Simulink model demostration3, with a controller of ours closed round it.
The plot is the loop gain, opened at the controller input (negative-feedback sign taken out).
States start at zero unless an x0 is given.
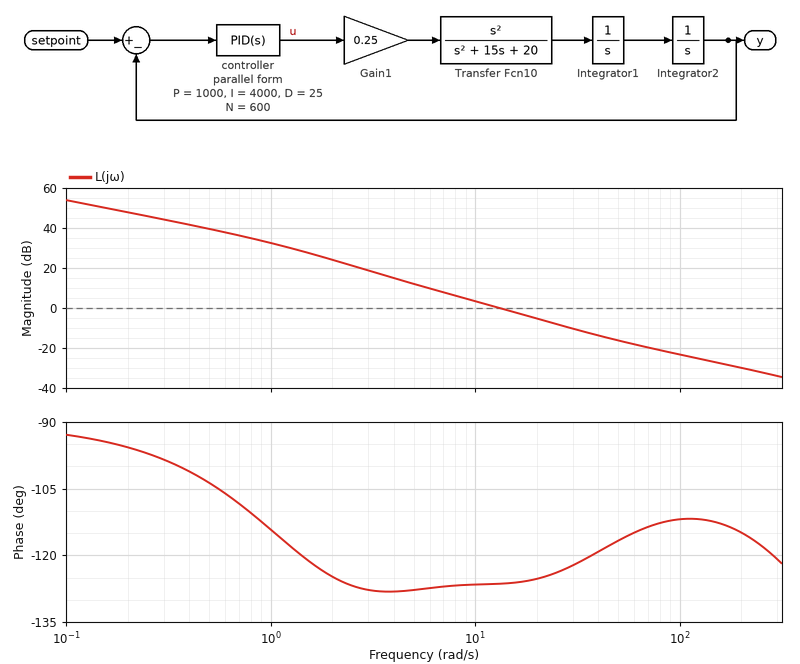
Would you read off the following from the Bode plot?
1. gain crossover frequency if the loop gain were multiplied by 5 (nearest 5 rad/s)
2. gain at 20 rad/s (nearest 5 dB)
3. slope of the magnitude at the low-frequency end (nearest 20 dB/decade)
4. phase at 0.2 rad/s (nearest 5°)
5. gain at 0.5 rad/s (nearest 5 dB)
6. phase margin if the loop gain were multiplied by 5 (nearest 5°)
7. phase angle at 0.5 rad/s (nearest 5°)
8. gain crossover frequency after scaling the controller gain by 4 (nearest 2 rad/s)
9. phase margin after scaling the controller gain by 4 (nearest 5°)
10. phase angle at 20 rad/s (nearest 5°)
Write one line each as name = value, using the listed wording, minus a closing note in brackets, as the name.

gain crossover frequency if the loop gain were multiplied by 5 = 40 rad/s
gain at 20 rad/s = -5 dB
slope of the magnitude at the low-frequency end = -20 dB/decade
phase at 0.2 rad/s = -95°
gain at 0.5 rad/s = 40 dB
phase margin if the loop gain were multiplied by 5 = 60°
phase angle at 0.5 rad/s = -105°
gain crossover frequency after scaling the controller gain by 4 = 34 rad/s
phase margin after scaling the controller gain by 4 = 60°
phase angle at 20 rad/s = -125°
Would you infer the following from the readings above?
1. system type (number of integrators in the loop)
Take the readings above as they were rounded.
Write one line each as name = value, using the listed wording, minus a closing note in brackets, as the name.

system type = 1
